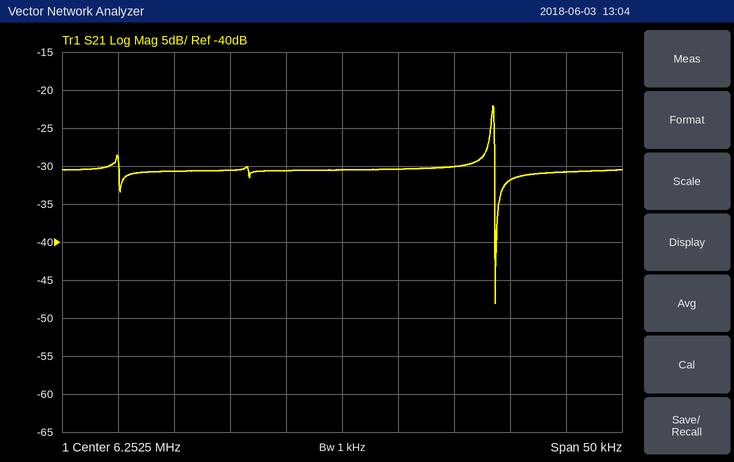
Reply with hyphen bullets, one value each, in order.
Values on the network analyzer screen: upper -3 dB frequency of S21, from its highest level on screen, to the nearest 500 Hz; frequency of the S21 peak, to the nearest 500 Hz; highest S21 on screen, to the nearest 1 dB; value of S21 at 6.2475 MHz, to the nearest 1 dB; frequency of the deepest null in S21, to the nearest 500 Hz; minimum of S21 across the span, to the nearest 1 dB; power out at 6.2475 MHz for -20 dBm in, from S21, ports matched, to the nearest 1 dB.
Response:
- 6.2660 MHz
- 6.2660 MHz
- -22 dB
- -31 dB
- 6.2660 MHz
- -48 dB
- -51 dBm
